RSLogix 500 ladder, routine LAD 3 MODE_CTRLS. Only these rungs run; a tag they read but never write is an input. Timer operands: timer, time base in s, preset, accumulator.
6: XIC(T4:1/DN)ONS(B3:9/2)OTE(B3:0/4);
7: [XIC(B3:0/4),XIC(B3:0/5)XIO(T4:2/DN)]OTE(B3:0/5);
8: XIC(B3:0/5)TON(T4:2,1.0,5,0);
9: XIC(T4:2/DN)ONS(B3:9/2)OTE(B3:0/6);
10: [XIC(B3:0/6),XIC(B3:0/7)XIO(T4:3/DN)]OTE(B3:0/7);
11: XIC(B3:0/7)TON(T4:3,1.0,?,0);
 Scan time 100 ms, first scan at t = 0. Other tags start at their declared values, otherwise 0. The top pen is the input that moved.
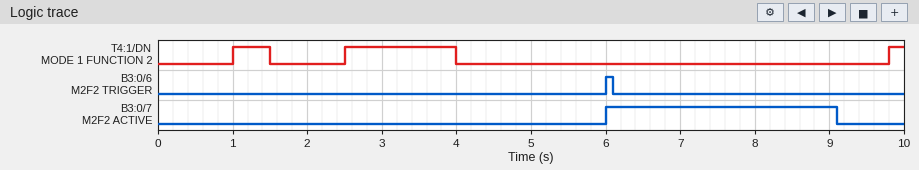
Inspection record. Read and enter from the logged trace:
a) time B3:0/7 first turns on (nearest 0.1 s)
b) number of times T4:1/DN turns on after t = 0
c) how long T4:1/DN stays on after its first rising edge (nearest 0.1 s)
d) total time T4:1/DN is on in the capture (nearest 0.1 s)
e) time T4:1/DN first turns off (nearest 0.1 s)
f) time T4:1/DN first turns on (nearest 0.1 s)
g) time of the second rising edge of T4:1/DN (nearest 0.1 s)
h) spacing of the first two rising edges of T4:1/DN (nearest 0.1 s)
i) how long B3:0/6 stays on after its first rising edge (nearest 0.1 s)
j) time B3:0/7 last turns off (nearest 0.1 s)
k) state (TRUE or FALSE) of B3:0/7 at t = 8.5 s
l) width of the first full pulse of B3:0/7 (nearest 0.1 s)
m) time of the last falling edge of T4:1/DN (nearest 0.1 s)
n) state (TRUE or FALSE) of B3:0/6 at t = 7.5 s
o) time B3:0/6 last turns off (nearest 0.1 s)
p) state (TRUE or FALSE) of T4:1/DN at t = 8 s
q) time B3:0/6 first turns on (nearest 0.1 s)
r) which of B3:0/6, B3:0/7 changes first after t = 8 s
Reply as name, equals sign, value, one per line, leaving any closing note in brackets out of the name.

time B3:0/7 first turns on = 6.0 s
number of times T4:1/DN turns on after t = 0 = 3
how long T4:1/DN stays on after its first rising edge = 0.5 s
total time T4:1/DN is on in the capture = 2.2 s
time T4:1/DN first turns off = 1.5 s
time T4:1/DN first turns on = 1.0 s
time of the second rising edge of T4:1/DN = 2.5 s
spacing of the first two rising edges of T4:1/DN = 1.5 s
how long B3:0/6 stays on after its first rising edge = 0.1 s
time B3:0/7 last turns off = 9.1 s
state (TRUE or FALSE) of B3:0/7 at t = 8.5 s = TRUE
width of the first full pulse of B3:0/7 = 3.1 s
time of the last falling edge of T4:1/DN = 4.0 s
state (TRUE or FALSE) of B3:0/6 at t = 7.5 s = FALSE
time B3:0/6 last turns off = 6.1 s
state (TRUE or FALSE) of T4:1/DN at t = 8 s = FALSE
time B3:0/6 first turns on = 6.0 s
which of B3:0/6, B3:0/7 changes first after t = 8 s = B3:0/7
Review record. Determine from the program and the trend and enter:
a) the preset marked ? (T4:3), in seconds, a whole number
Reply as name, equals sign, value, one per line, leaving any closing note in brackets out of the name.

the preset marked ? (T4:3), in seconds, a whole number = 3 s
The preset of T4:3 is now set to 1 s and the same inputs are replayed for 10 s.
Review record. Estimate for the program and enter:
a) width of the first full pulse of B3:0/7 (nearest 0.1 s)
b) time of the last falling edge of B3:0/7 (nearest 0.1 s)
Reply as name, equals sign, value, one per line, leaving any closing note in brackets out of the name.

width of the first full pulse of B3:0/7 = 1.1 s
time of the last falling edge of B3:0/7 = 7.1 s
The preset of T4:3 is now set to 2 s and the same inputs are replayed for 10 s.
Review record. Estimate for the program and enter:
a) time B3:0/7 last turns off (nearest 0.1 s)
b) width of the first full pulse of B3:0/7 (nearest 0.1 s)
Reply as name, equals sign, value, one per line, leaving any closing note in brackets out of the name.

time B3:0/7 last turns off = 8.1 s
width of the first full pulse of B3:0/7 = 2.1 s
